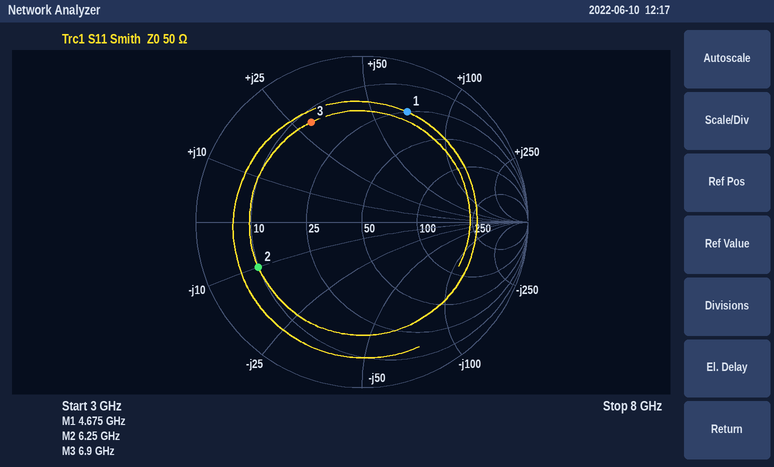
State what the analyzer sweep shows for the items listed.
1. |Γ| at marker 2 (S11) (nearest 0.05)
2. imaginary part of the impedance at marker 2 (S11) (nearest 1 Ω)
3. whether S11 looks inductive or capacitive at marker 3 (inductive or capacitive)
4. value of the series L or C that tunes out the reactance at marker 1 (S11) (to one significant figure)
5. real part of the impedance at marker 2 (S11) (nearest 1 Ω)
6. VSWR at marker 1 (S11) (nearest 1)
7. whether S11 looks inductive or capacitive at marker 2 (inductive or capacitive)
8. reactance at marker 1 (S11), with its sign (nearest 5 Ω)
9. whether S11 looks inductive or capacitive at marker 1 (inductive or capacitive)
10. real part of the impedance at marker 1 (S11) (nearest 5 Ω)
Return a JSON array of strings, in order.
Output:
["0.70", "-10 Ω", "inductive", "500 fF", "10 Ω", "6", "capacitive", "+70 Ω", "inductive", "25 Ω"]
